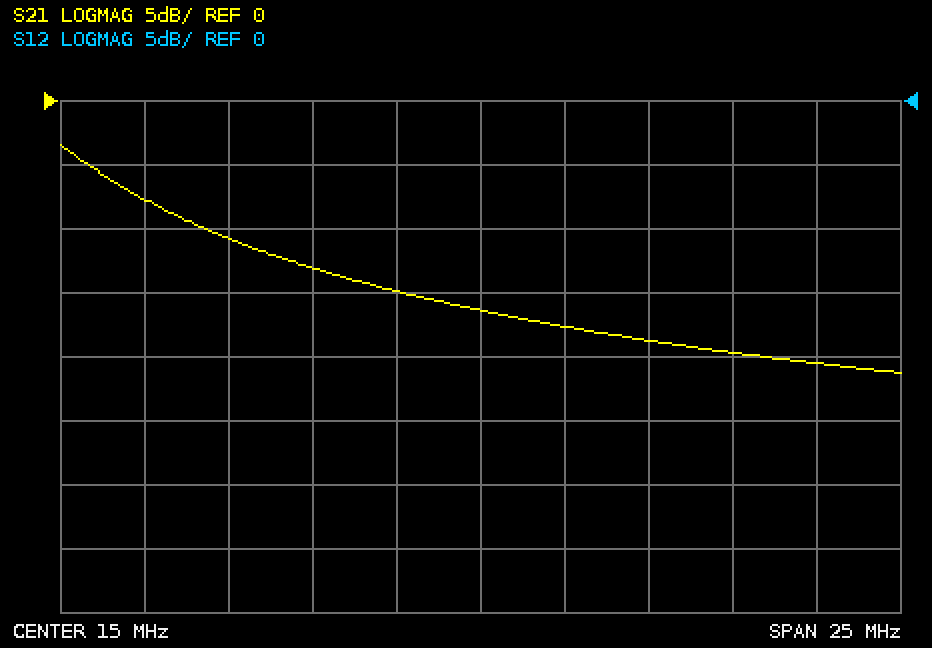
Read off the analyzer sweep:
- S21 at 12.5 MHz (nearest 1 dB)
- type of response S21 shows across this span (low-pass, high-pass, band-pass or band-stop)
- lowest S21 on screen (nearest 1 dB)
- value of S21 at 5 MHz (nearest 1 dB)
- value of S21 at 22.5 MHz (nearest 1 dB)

-15 dB
low-pass
-21 dB
-8 dB
-20 dB
